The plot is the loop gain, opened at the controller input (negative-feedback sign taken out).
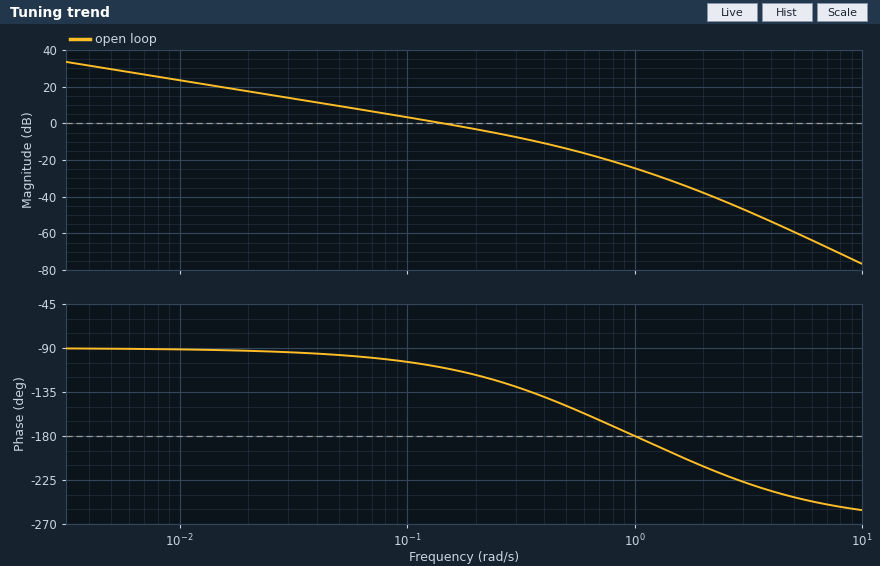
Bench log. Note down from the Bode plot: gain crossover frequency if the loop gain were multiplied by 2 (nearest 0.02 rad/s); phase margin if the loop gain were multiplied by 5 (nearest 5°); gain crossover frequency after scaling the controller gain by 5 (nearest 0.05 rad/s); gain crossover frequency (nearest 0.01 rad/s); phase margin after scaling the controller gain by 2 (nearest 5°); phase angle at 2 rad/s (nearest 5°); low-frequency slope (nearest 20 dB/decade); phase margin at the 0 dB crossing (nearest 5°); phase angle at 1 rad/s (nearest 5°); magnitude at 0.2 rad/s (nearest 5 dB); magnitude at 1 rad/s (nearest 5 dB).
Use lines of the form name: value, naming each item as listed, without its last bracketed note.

gain crossover frequency if the loop gain were multiplied by 2: 0.26 rad/s
phase margin if the loop gain were multiplied by 5: 30°
gain crossover frequency after scaling the controller gain by 5: 0.50 rad/s
gain crossover frequency: 0.14 rad/s
phase margin after scaling the controller gain by 2: 55°
phase angle at 2 rad/s: -210°
low-frequency slope: -20 dB/decade
phase margin at the 0 dB crossing: 70°
phase angle at 1 rad/s: -180°
magnitude at 0.2 rad/s: -5 dB
magnitude at 1 rad/s: -25 dB
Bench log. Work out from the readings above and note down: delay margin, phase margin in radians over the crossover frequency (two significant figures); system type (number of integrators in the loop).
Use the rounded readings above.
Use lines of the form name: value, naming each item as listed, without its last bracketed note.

delay margin, phase margin in radians over the crossover frequency: 8.7 s
system type: 1
